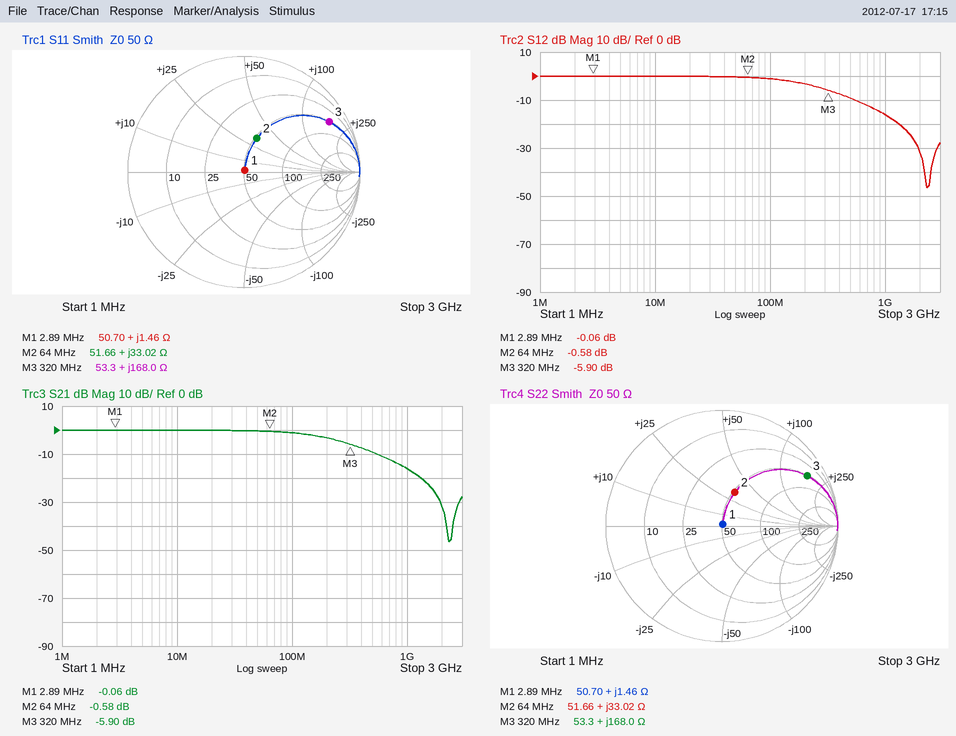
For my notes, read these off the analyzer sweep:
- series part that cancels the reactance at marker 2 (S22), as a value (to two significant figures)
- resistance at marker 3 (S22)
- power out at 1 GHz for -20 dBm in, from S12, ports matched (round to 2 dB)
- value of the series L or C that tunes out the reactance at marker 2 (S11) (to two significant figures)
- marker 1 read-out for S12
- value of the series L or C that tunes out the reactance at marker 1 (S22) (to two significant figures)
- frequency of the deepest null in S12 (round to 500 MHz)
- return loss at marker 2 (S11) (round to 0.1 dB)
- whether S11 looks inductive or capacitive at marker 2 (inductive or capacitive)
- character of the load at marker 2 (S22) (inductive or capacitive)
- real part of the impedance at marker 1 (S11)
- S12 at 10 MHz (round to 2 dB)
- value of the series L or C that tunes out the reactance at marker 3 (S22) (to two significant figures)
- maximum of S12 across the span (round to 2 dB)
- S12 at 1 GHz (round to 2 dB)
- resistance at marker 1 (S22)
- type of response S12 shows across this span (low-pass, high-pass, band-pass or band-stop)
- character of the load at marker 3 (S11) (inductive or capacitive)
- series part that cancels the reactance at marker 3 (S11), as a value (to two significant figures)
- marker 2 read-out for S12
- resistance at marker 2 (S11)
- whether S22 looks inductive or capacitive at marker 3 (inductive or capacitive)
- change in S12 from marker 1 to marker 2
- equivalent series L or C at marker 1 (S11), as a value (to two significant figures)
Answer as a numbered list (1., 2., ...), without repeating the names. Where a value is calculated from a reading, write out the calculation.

1. C = 1/(2π × 64 MHz × 33.02 Ω) ≈ 75 pF
2. 53.3 Ω
3. -20 dBm + (-16 dB) = -36 dBm
4. C = 1/(2π × 64 MHz × 33.02 Ω) ≈ 75 pF
5. -0.06 dB
6. C = 1/(2π × 2.89 MHz × 1.46 Ω) ≈ 38 nF
7. 2.5 GHz
8. 10.2 dB
9. inductive
10. inductive
11. 50.70 Ω
12. 0 dB
13. C = 1/(2π × 320 MHz × 168 Ω) ≈ 3.0 pF
14. 0 dB
15. -16 dB
16. 50.70 Ω
17. low-pass
18. inductive
19. C = 1/(2π × 320 MHz × 168 Ω) ≈ 3.0 pF
20. -0.58 dB
21. 51.66 Ω
22. inductive
23. -0.58 − (-0.06) = -0.52 dB
24. L = 1.46 Ω/(2π × 2.89 MHz) ≈ 80 nH
